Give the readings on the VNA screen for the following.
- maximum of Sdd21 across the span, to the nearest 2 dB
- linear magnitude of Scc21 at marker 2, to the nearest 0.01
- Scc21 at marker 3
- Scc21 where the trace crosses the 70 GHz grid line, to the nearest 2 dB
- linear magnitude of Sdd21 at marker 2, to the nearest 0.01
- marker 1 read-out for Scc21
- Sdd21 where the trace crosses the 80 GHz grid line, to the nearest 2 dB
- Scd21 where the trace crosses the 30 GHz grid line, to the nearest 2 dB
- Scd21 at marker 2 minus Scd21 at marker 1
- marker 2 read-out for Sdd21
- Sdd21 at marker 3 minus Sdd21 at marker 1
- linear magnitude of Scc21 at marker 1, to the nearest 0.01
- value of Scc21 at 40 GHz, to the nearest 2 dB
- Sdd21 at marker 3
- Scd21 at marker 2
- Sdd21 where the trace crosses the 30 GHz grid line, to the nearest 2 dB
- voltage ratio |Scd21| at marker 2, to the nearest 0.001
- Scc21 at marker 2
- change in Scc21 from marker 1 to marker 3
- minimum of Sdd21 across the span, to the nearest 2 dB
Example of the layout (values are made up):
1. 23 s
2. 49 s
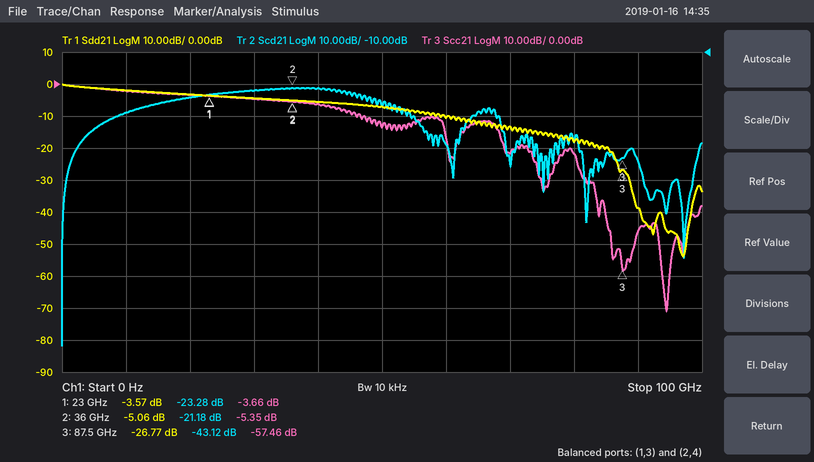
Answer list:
1. 0 dB
2. 0.54
3. -57.46 dB
4. -22 dB
5. 0.56
6. -3.66 dB
7. -18 dB
8. -22 dB
9. 2.10 dB
10. -5.06 dB
11. -23.20 dB
12. 0.66
13. -6 dB
14. -26.77 dB
15. -21.18 dB
16. -4 dB
17. 0.087
18. -5.35 dB
19. -53.80 dB
20. -54 dB
